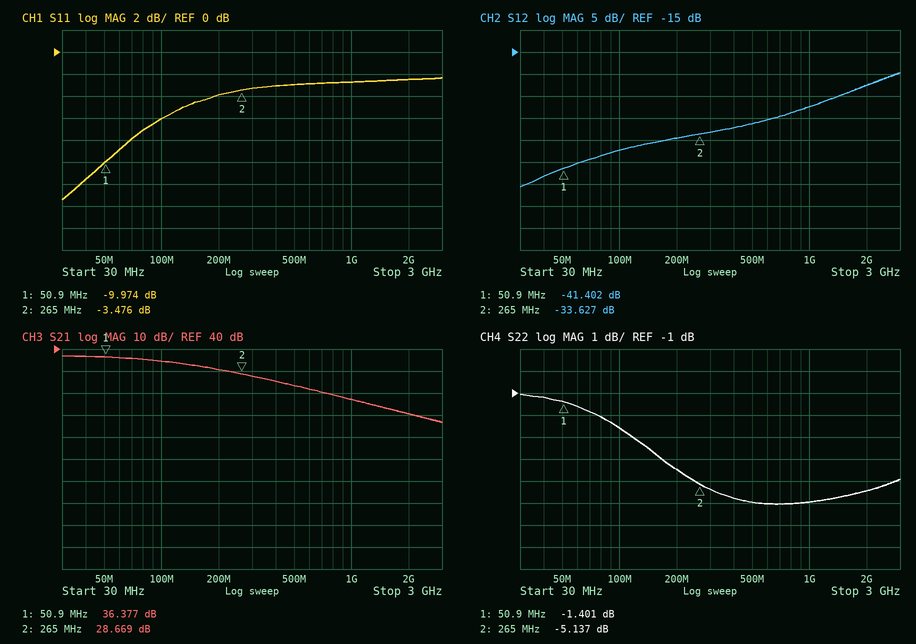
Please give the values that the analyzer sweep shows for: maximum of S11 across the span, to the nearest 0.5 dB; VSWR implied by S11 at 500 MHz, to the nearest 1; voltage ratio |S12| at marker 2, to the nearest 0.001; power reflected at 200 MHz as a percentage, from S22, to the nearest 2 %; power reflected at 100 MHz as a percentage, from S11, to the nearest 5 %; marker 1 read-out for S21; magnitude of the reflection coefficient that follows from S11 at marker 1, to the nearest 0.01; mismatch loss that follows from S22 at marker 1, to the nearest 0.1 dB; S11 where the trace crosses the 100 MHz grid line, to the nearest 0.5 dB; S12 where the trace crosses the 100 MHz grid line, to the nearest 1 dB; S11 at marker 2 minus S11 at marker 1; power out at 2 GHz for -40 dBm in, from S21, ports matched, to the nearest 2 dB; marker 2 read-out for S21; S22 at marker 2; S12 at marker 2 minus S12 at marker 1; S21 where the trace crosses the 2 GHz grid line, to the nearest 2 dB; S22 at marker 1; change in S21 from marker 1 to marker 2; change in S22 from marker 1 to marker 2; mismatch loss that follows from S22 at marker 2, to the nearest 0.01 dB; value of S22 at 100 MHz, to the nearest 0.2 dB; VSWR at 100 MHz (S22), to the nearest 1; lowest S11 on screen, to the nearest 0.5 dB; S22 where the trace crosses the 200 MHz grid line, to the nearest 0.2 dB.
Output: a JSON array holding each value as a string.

["-2.5 dB", "6", "0.021", "36 %", "25 %", "36.377 dB", "0.32", "5.6 dB", "-6.0 dB", "-37 dB", "6.498 dB", "-30 dBm", "28.669 dB", "-5.137 dB", "7.775 dB", "10 dB", "-1.401 dB", "-7.708 dB", "-3.736 dB", "1.59 dB", "-2.6 dB", "7", "-13.5 dB", "-4.4 dB"]
